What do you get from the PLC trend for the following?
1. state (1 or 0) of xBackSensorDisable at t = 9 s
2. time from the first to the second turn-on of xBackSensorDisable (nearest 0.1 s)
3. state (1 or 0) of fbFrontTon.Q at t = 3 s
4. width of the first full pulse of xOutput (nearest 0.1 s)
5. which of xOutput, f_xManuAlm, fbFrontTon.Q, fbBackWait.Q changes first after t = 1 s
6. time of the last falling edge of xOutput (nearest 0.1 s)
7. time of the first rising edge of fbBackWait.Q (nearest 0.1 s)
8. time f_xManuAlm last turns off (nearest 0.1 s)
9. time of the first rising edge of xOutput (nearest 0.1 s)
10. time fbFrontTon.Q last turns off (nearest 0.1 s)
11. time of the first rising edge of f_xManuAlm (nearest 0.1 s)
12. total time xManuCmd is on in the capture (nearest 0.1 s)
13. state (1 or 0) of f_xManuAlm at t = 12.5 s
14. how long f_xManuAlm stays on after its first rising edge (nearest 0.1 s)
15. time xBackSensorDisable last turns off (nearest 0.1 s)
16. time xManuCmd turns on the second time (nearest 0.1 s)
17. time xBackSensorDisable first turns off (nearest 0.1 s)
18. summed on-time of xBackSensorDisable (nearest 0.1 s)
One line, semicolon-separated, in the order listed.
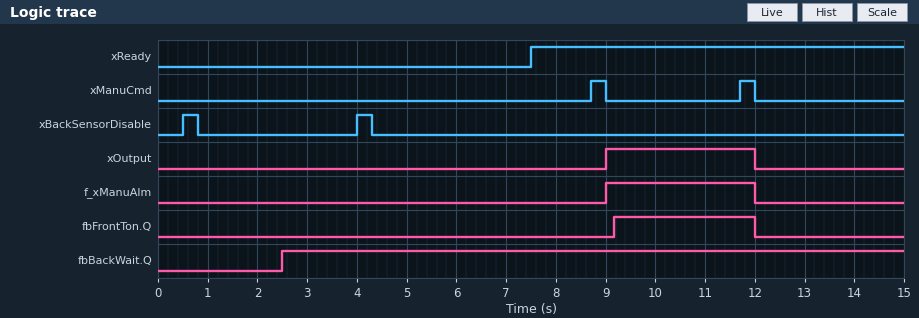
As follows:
0; 3.5 s; 0; 3.0 s; fbBackWait.Q; 12.0 s; 2.5 s; 12.0 s; 9.0 s; 12.0 s; 9.0 s; 0.6 s; 0; 3.0 s; 4.3 s; 11.7 s; 0.8 s; 0.6 s
